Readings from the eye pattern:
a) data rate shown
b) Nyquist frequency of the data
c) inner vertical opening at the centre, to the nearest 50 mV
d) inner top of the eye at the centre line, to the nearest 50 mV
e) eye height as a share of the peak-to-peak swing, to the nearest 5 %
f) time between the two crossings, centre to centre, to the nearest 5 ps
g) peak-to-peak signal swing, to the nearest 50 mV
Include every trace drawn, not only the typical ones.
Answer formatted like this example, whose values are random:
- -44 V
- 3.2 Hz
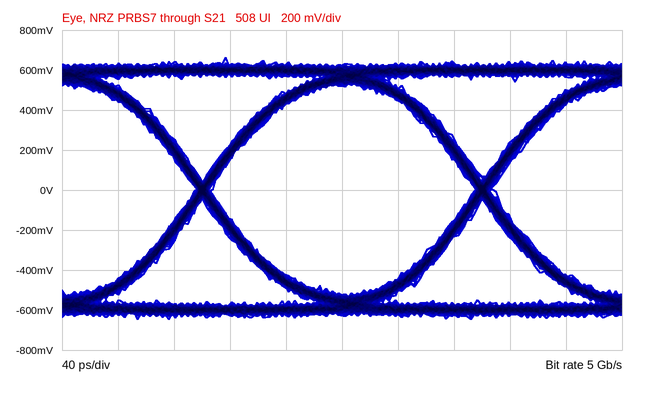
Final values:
- 5 Gb/s
- 2.5 GHz
- 1.05 V
- 500 mV
- 80 %
- 200 ps
- 1.30 V
